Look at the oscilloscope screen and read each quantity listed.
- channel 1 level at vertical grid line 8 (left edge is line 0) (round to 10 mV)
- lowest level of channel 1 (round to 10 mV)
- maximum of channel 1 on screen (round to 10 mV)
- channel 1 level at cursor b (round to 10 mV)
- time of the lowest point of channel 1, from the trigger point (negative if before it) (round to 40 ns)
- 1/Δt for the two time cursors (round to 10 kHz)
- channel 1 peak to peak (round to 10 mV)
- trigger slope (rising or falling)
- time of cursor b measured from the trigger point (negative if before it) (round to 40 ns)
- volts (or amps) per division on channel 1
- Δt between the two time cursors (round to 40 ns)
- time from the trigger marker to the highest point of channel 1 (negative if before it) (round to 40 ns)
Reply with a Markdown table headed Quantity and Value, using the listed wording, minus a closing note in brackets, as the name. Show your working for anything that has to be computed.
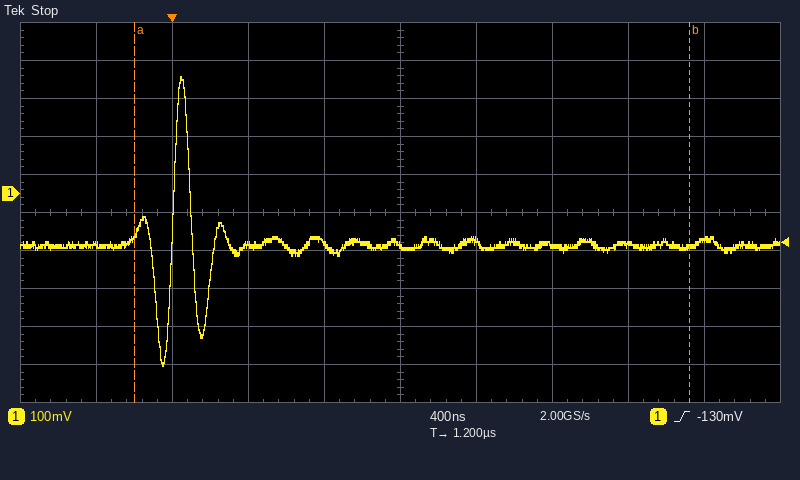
| Quantity | Value |
|---|---|
| channel 1 level at vertical grid line 8 (left edge is line 0) | -130 mV |
| lowest level of channel 1 | -450 mV |
| maximum of channel 1 on screen | 310 mV |
| channel 1 level at cursor b | -140 mV |
| time of the lowest point of channel 1, from the trigger point (negative if before it) | -40 ns |
| 1/Δt for the two time cursors | 1 / 2.92 µs ≈ 340 kHz |
| channel 1 peak to peak | 310 mV − (-450 mV) = 760 mV |
| trigger slope | rising |
| time of cursor b measured from the trigger point (negative if before it) | +2.72 µs |
| volts (or amps) per division on channel 1 | 100 mV |
| Δt between the two time cursors | 2.92 µs |
| time from the trigger marker to the highest point of channel 1 (negative if before it) | +40 ns |
